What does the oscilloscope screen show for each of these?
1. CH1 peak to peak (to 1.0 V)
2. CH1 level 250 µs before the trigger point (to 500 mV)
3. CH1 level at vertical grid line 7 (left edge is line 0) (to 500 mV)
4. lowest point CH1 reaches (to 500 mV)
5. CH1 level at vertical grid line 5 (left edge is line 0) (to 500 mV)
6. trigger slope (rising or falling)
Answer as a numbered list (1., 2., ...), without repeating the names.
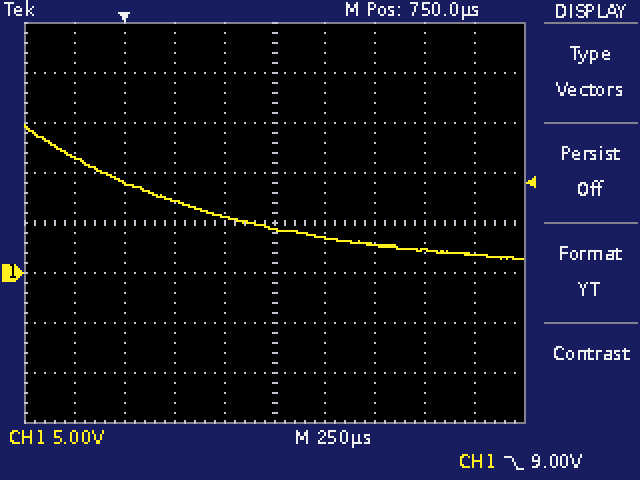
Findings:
1. 13.0 V
2. 11.5 V
3. 3.0 V
4. 1.5 V
5. 4.5 V
6. falling
